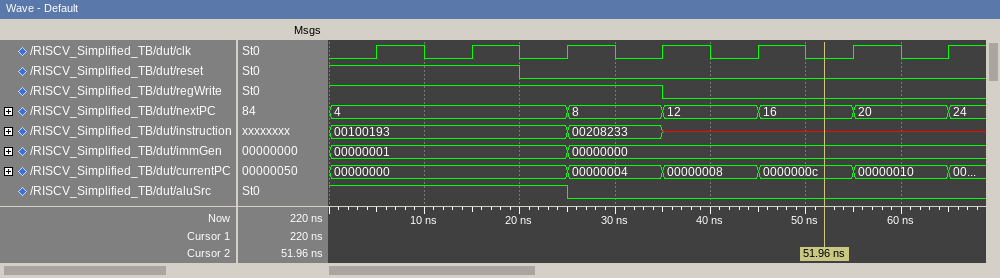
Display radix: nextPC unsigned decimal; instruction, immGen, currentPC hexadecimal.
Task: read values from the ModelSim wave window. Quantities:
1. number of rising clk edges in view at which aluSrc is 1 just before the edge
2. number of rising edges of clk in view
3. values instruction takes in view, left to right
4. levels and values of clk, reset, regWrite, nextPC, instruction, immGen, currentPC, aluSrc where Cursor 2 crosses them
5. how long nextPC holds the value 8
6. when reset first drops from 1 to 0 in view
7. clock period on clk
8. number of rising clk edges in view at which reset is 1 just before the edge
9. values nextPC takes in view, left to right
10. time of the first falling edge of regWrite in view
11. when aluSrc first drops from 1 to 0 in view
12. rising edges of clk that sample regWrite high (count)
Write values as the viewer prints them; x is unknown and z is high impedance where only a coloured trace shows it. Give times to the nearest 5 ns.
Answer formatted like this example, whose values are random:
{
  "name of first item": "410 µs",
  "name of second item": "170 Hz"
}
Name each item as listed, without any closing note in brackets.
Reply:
{
  "number of rising clk edges in view at which aluSrc is 1 just before the edge": "3",
  "number of rising edges of clk in view": "7",
  "values instruction takes in view, left to right": "00100193, 00208233, x",
  "levels and values of clk, reset, regWrite, nextPC, instruction, immGen, currentPC, aluSrc where Cursor 2 crosses them": "clk=0, reset=0, regWrite=0, nextPC=16, instruction=x, immGen=00000000, currentPC=0000000c, aluSrc=0",
  "how long nextPC holds the value 8": "10 ns",
  "when reset first drops from 1 to 0 in view": "20 ns",
  "clock period on clk": "10 ns",
  "number of rising clk edges in view at which reset is 1 just before the edge": "2",
  "values nextPC takes in view, left to right": "4, 8, 12, 16, 20, 24",
  "time of the first falling edge of regWrite in view": "35 ns",
  "when aluSrc first drops from 1 to 0 in view": "25 ns",
  "rising edges of clk that sample regWrite high": "4"
}
